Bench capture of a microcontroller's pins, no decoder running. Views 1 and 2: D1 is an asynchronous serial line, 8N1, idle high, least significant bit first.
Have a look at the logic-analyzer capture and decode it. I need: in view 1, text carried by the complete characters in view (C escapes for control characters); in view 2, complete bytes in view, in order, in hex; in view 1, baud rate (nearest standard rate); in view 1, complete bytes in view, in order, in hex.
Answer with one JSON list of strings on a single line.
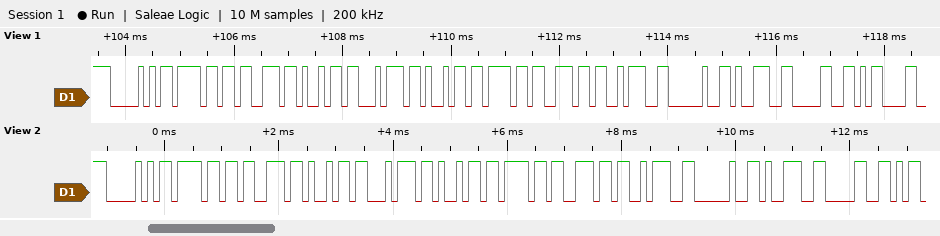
["\"Position: 90\\r\"", "50 6F 73 69 74 69 6F 6E 3A 20 39 30", "9600 baud", "0x50 0x6F 0x73 0x69 0x74 0x69 0x6F 0x6E 0x3A 0x20 0x39 0x30 0x0D"]
